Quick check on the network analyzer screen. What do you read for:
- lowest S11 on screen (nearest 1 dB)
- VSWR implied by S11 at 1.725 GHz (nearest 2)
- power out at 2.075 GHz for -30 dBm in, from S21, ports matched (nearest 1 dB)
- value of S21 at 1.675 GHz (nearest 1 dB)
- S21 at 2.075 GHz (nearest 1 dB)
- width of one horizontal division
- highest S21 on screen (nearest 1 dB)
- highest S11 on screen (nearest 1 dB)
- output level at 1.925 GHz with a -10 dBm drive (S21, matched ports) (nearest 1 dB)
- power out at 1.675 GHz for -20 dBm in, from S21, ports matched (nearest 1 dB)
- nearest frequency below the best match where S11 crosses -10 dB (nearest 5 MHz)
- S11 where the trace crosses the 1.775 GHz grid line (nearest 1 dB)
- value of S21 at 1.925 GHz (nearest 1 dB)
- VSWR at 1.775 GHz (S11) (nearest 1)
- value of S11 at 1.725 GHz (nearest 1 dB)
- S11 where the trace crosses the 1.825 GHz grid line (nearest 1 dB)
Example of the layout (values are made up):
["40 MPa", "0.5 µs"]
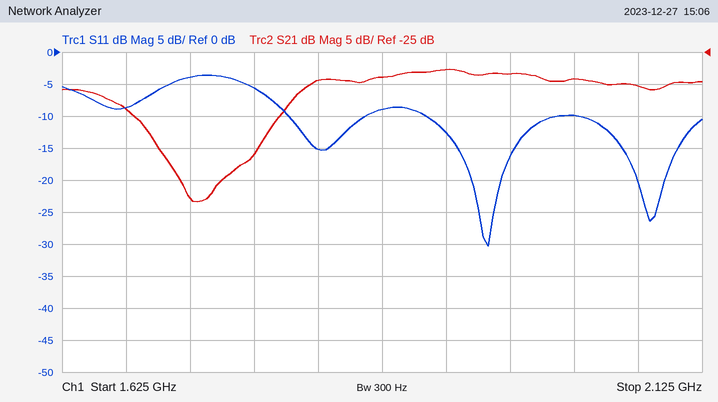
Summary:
["-30 dB", "4", "-60 dBm", "-34 dB", "-30 dB", "50 MHz", "-28 dB", "-4 dB", "-38 dBm", "-54 dBm", "1.910 GHz", "-6 dB", "-28 dB", "3", "-4 dB", "-15 dB"]
